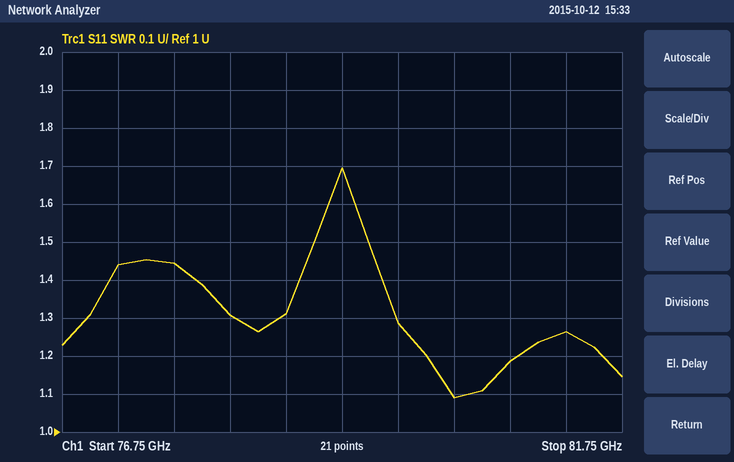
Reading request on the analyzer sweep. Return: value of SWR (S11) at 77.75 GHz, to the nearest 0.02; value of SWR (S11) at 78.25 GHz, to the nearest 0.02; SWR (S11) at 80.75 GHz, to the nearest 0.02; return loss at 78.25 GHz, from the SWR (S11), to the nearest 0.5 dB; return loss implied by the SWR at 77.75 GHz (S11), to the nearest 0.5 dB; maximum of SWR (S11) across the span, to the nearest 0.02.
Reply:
1.44
1.30
1.18
17.5 dB
15.0 dB
1.70
